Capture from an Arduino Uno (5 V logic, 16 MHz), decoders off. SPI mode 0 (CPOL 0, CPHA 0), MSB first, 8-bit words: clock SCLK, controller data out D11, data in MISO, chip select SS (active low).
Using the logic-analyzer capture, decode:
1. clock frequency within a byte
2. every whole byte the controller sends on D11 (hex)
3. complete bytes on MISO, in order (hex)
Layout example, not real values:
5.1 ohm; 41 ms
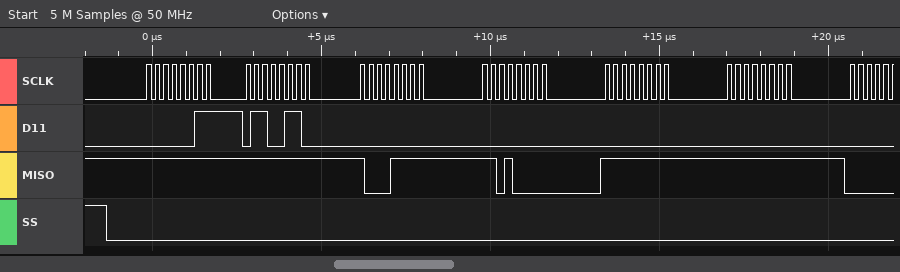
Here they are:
4 MHz; 03 66 00 00 00 00; FF FF 8F D0 FF FF
